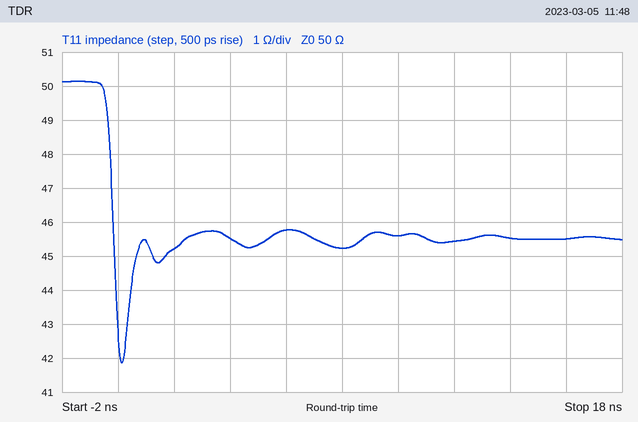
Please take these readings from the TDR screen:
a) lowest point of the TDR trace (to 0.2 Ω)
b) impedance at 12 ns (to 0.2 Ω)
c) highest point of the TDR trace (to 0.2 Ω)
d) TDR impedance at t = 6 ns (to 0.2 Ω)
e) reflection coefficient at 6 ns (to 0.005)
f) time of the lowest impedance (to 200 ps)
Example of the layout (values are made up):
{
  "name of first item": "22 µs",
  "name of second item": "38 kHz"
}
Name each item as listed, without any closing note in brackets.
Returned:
{
  "lowest point of the TDR trace": "41.8 Ω",
  "impedance at 12 ns": "45.4 Ω",
  "highest point of the TDR trace": "50.2 Ω",
  "TDR impedance at t = 6 ns": "45.8 Ω",
  "reflection coefficient at 6 ns": "-0.045",
  "time of the lowest impedance": "200 ps"
}
